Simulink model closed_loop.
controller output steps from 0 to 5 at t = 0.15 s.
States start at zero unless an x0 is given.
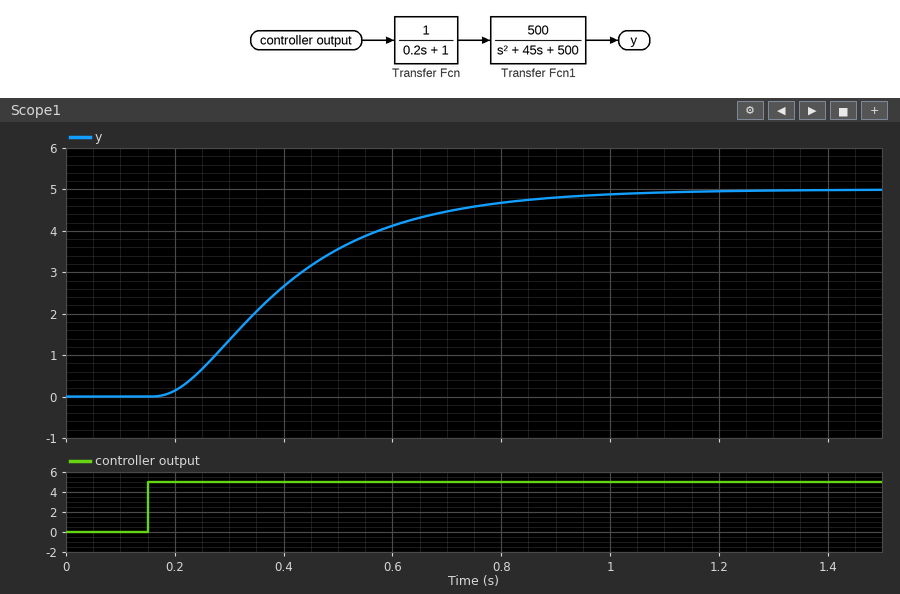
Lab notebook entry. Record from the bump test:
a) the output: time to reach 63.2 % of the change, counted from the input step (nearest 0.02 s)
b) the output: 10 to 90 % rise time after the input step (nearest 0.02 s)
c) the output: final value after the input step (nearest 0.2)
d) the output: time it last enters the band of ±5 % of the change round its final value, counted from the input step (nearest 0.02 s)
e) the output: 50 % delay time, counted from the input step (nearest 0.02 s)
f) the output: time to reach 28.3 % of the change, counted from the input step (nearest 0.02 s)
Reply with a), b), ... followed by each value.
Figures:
a) 0.30 s
b) 0.48 s
c) 5.0
d) 0.70 s
e) 0.24 s
f) 0.16 s
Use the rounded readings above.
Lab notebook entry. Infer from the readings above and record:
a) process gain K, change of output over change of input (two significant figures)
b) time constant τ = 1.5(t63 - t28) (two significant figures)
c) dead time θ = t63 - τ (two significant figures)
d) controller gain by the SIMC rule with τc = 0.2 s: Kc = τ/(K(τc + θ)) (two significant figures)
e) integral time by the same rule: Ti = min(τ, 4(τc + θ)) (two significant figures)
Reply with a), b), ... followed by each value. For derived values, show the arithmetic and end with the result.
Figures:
a) (5 - 0) / 5 = 1.0
b) 1.5 × (0.3 - 0.16) = 0.21 s
c) 0.3 - 0.21 = 0.090 s
d) 0.21 / (1 × (0.2 + 0.09)) = 0.72
e) min(0.21, 4 × (0.2 + 0.09)) = 0.21 s
